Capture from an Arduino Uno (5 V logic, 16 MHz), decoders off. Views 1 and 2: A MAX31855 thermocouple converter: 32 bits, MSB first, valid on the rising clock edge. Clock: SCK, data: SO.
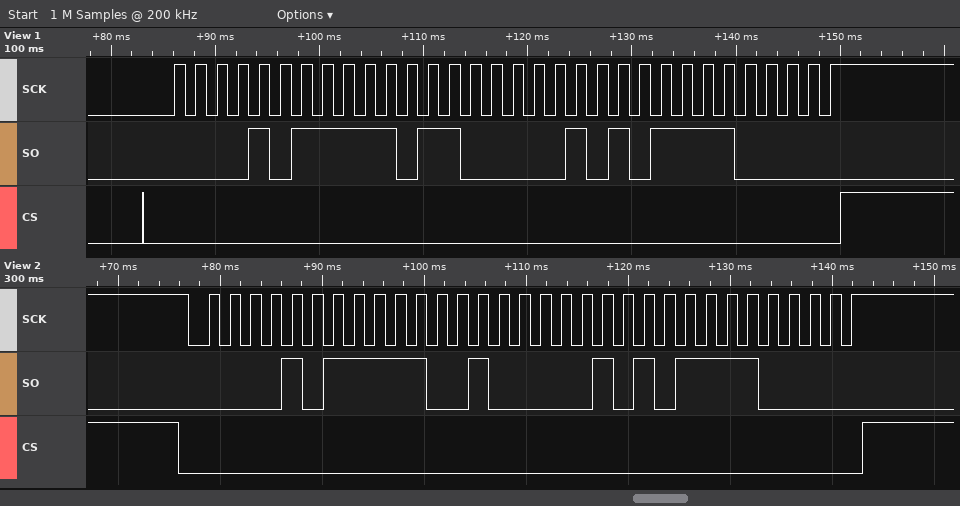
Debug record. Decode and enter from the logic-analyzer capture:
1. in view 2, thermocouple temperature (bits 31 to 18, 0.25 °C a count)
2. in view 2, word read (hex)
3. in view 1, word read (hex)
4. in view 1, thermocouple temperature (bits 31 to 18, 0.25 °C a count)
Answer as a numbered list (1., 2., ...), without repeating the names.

1. 190.25 °C
2. 0x0BE415E0
3. 0x0BEC15E0
4. 190.75 °C
